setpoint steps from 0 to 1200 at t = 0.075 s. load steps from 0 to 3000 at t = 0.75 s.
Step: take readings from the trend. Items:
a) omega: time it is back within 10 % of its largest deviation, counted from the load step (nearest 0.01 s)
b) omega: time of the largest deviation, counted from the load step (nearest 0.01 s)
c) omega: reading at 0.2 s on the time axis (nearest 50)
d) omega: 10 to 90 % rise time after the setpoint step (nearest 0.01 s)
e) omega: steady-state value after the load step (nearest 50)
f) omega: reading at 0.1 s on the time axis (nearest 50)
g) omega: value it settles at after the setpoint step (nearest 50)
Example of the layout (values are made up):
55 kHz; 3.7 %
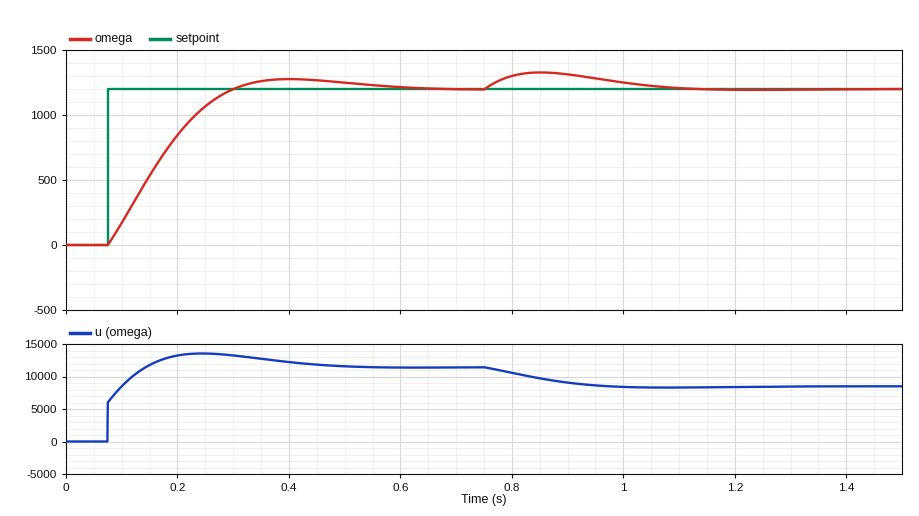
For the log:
0.33 s; 0.10 s; 850; 0.16 s; 1200; 150; 1200
